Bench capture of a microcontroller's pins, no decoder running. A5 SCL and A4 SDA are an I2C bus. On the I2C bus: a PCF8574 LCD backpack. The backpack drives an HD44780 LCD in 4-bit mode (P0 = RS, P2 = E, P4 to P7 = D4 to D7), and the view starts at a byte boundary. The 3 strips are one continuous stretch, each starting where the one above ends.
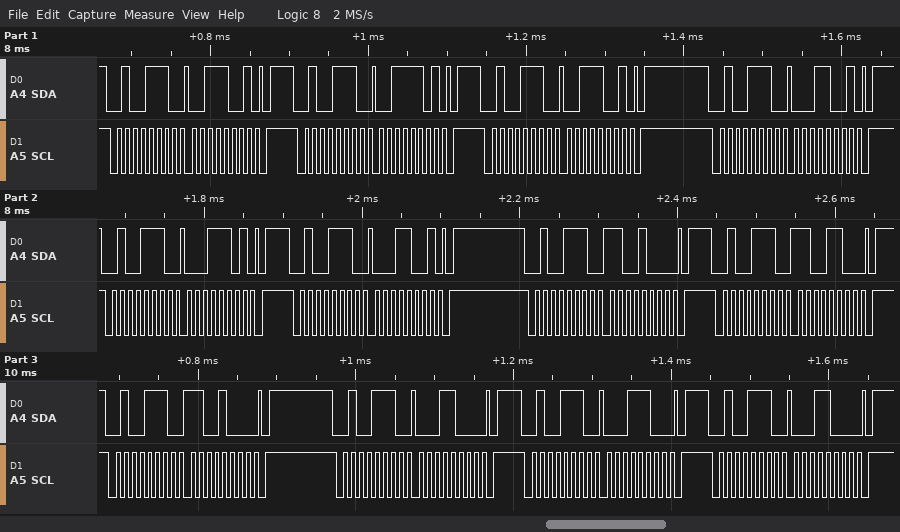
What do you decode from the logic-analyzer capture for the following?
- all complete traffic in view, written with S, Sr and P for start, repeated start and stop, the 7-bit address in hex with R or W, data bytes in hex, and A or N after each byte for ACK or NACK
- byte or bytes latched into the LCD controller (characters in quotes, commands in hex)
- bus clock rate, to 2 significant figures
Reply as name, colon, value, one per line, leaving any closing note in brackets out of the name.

all complete traffic in view, written with S, Sr and P for start, repeated start and stop, the 7-bit address in hex with R or W, data bytes in hex, and A or N after each byte for ACK or NACK: S 27W A 39 A P S 27W A 3D A P S 27W A 39 A P S 27W A 19 A P S 27W A 1D A P S 27W A 19 A P S 27W A C8 A P S 27W A CC A P S 27W A C8 A P S 27W A 18 A P S 27W A 1C A P S 27W A 18 A P
byte or bytes latched into the LCD controller: '1' 0xC1
bus clock rate, to 2 significant figures: 100 kHz
